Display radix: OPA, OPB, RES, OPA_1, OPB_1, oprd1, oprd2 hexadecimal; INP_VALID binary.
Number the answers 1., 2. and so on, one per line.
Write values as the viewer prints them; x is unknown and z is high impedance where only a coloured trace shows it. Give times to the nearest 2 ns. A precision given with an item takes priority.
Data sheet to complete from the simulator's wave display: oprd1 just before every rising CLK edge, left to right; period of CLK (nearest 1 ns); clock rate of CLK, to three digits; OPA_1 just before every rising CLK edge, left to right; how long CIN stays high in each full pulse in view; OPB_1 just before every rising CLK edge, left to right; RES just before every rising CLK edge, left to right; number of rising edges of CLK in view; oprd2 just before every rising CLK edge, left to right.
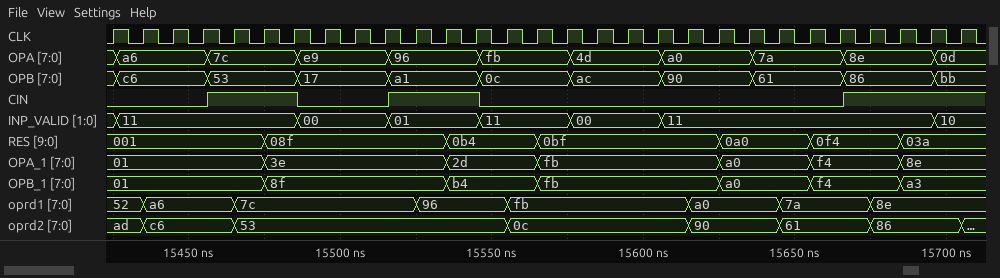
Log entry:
1. 52, 52, a6, a6, a6, 7c, 7c, 7c, 7c, 7c, 7c, 96, 96, 96, fb, fb, fb, fb, fb, fb, a0, a0, a0, 7a, 7a, 7a, 8e, 8e, 8e
2. 10 ns
3. 100 MHz
4. 01, 01, 01, 01, 01, 01, 3e, 3e, 3e, 3e, 3e, 3e, 2d, 2d, 2d, fb, fb, fb, fb, fb, fb, a0, a0, a0, f4, f4, f4, 8e, 8e
5. 30 ns, 30 ns
6. 01, 01, 01, 01, 01, 01, 8f, 8f, 8f, 8f, 8f, 8f, b4, b4, b4, fb, fb, fb, fb, fb, fb, a0, a0, a0, f4, f4, f4, a3, a3
7. 001, 001, 001, 001, 001, 001, 08f, 08f, 08f, 08f, 08f, 08f, 0b4, 0b4, 0b4, 0bf, 0bf, 0bf, 0bf, 0bf, 0bf, 0a0, 0a0, 0a0, 0f4, 0f4, 0f4, 03a, 03a
8. 29
9. ad, ad, c6, c6, c6, 53, 53, 53, 53, 53, 53, 53, 53, 53, 0c, 0c, 0c, 0c, 0c, 0c, 90, 90, 90, 61, 61, 61, 86, 86, 86
